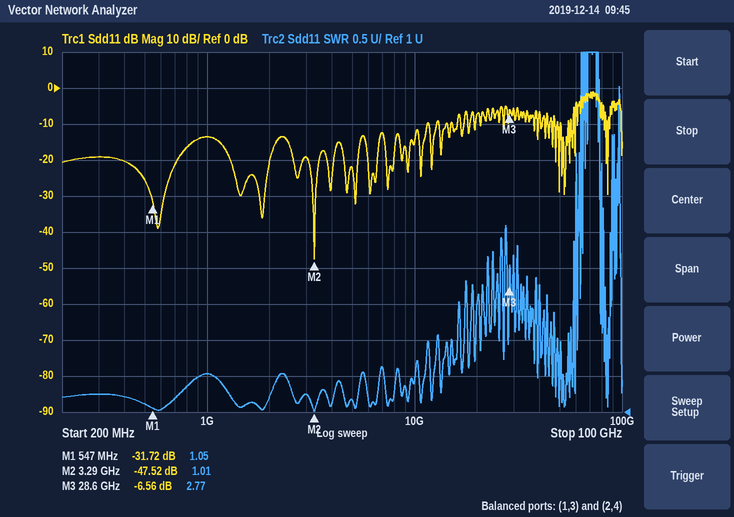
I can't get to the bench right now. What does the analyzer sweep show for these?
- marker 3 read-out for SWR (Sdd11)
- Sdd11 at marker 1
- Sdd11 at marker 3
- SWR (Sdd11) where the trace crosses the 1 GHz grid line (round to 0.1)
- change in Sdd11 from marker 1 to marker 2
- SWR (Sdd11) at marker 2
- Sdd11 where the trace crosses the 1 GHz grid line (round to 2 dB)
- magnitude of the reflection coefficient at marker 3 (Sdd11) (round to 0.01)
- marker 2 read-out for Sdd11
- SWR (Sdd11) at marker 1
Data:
2.77
-31.72 dB
-6.56 dB
1.5
-15.80 dB
1.01
-14 dB
0.47
-47.52 dB
1.05
